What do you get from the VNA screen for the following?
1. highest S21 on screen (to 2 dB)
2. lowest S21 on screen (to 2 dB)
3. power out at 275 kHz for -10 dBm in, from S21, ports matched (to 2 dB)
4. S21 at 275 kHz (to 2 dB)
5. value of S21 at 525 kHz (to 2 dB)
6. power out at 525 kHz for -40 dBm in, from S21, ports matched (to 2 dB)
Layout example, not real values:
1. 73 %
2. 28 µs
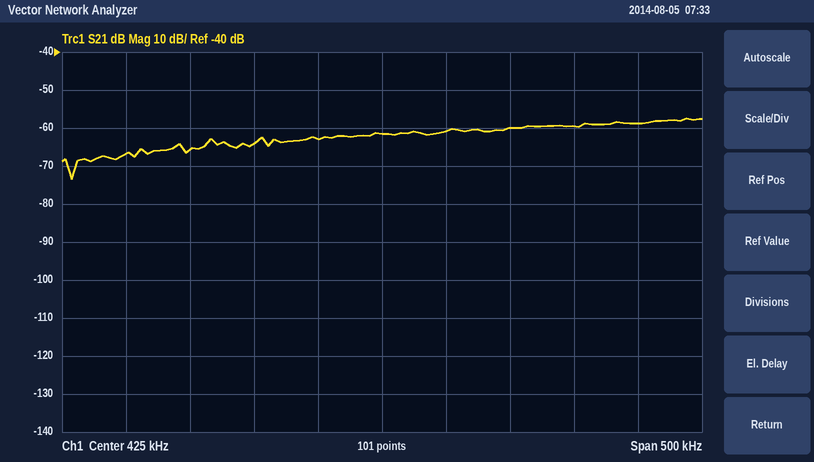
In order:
1. -58 dB
2. -74 dB
3. -76 dBm
4. -66 dB
5. -60 dB
6. -100 dBm
